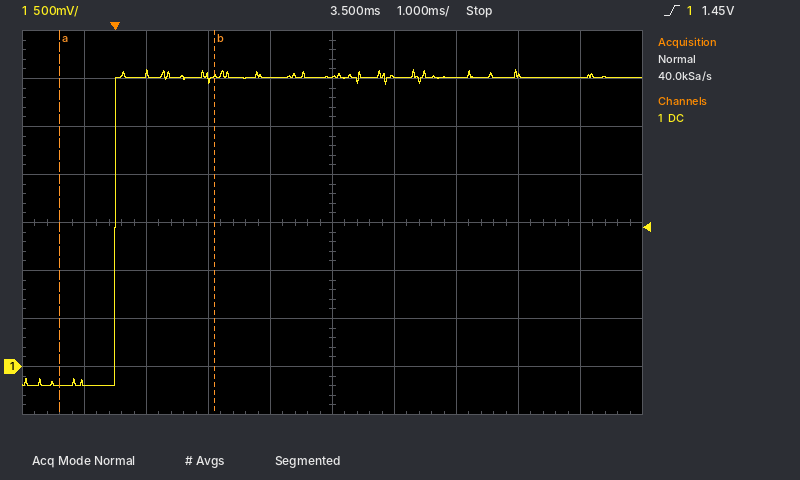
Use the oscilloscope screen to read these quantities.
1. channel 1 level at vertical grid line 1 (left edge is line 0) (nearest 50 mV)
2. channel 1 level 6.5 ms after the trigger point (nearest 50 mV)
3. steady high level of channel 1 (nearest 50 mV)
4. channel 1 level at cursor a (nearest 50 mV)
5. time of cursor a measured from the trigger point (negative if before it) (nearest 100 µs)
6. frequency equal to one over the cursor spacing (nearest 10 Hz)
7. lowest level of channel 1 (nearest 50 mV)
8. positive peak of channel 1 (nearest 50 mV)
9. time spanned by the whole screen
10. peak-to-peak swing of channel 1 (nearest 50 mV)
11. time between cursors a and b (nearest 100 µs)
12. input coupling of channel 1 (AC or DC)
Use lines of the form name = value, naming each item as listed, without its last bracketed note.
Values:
channel 1 level at vertical grid line 1 (left edge is line 0) = -150 mV
channel 1 level 6.5 ms after the trigger point = 3.05 V
steady high level of channel 1 = 3.00 V
channel 1 level at cursor a = -200 mV
time of cursor a measured from the trigger point (negative if before it) = -900 µs
frequency equal to one over the cursor spacing = 400 Hz
lowest level of channel 1 = -200 mV
positive peak of channel 1 = 3.10 V
time spanned by the whole screen = 10 ms
peak-to-peak swing of channel 1 = 3.30 V
time between cursors a and b = 2.5 ms
input coupling of channel 1 = DC
